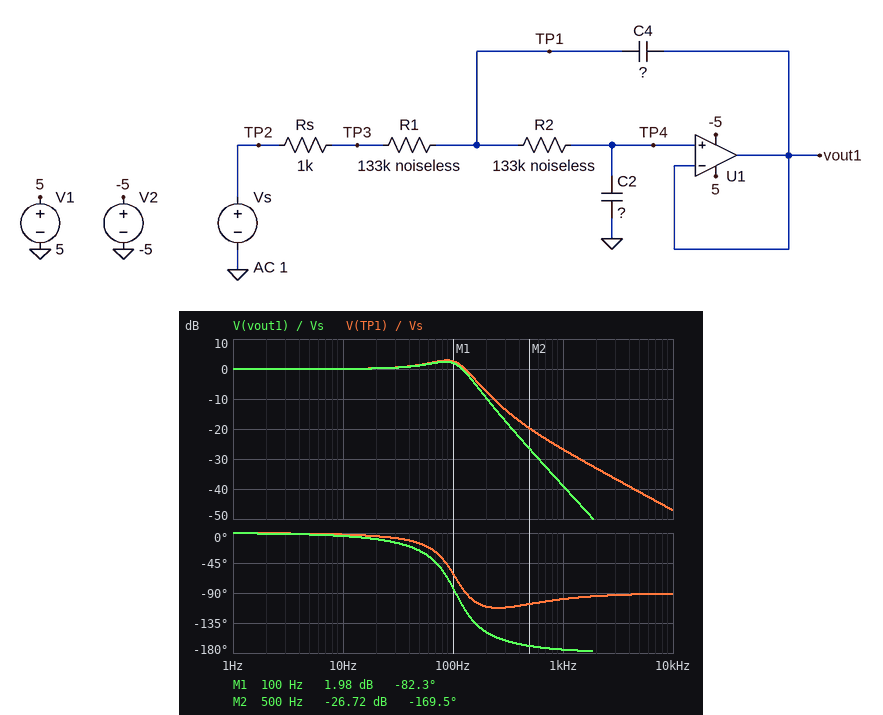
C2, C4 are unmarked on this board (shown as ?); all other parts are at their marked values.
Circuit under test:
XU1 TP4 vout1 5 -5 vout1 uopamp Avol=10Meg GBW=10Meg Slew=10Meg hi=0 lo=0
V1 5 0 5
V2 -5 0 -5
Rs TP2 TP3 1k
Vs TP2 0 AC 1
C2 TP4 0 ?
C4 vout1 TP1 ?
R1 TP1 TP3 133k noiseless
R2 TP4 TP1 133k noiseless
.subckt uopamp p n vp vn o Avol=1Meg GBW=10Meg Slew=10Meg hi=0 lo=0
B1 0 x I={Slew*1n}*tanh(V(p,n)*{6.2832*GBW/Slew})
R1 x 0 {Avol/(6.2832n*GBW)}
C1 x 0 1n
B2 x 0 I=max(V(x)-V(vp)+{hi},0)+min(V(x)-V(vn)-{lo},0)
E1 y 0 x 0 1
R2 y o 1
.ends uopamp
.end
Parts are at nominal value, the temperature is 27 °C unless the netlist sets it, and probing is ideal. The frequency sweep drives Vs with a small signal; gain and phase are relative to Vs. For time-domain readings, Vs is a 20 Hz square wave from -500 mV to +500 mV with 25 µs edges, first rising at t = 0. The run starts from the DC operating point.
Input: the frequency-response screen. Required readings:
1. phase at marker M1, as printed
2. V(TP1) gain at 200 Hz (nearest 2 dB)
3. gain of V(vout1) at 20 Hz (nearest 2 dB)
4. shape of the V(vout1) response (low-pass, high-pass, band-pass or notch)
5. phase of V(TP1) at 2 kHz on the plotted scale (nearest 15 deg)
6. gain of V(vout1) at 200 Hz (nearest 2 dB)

-82.3 deg
-8 dB
0 dB
low-pass
-90 deg
-10 dB
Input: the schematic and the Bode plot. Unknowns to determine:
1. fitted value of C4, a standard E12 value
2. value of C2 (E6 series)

27 nF
4.7 nF
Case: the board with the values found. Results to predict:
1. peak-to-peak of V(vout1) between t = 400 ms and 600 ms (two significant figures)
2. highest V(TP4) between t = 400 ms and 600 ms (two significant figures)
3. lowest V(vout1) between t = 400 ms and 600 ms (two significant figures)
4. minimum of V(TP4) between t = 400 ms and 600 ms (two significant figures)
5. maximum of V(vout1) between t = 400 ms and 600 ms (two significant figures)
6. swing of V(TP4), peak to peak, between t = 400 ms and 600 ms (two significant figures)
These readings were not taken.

1.5 V
740 mV
-740 mV
-740 mV
740 mV
1.5 V
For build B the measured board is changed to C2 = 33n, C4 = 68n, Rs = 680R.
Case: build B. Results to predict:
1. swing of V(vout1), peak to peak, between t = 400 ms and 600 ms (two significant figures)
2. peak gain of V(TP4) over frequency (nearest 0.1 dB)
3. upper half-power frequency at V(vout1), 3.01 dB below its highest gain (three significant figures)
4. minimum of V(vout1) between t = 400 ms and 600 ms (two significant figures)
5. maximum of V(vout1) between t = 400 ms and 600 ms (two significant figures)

1.1 V
0 dB
25.6 Hz
-540 mV
540 mV
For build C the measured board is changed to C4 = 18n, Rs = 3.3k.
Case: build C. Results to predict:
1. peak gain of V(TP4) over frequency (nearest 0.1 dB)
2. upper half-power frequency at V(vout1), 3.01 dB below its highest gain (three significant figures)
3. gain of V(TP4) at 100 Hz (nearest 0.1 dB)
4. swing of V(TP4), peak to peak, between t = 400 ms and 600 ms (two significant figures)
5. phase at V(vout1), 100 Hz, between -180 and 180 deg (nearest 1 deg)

1.1 dB
150 Hz
1.0 dB
1.3 V
-64 deg
